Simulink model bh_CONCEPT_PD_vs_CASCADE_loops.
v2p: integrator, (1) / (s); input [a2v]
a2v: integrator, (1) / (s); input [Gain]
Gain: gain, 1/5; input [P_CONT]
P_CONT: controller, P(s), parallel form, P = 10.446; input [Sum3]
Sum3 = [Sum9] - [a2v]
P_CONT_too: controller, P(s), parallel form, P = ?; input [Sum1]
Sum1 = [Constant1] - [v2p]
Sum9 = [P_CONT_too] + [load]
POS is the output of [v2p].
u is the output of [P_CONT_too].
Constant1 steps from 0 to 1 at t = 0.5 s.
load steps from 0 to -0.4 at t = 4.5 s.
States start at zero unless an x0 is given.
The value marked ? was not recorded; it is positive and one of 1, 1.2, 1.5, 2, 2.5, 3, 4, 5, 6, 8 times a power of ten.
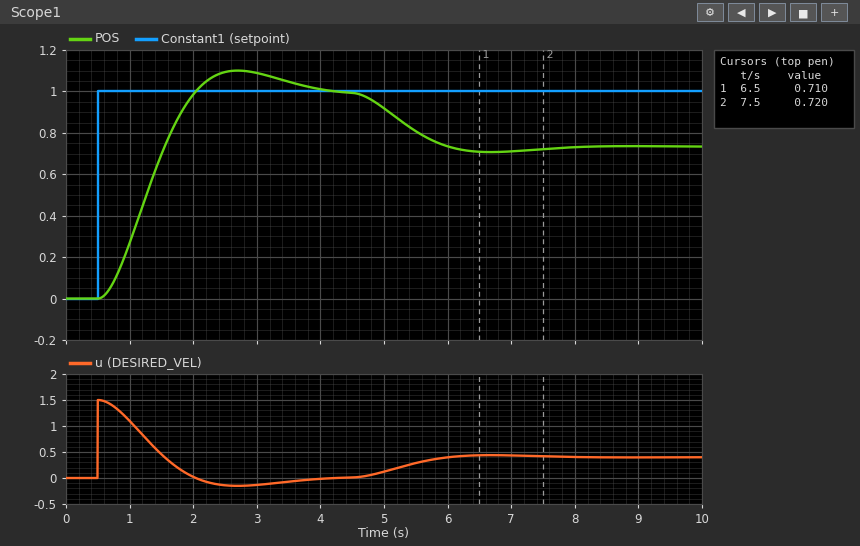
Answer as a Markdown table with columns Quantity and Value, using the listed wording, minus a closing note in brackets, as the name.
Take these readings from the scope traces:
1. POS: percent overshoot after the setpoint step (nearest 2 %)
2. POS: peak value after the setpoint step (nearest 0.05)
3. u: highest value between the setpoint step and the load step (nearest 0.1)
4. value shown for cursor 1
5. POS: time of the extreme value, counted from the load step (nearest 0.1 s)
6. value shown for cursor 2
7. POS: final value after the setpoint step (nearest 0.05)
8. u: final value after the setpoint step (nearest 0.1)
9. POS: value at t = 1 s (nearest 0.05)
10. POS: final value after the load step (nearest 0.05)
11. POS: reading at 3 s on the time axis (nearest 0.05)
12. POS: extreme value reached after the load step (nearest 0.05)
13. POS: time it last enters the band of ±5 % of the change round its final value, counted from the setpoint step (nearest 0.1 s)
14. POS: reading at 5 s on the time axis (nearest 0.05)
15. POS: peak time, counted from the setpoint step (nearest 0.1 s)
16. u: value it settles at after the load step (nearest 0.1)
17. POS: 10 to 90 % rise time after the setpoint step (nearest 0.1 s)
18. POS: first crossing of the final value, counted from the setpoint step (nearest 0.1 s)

| Quantity | Value |
|---|---|
| POS: percent overshoot after the setpoint step | 10 % |
| POS: peak value after the setpoint step | 1.10 |
| u: highest value between the setpoint step and the load step | 1.5 |
| value shown for cursor 1 | 0.710 |
| POS: time of the extreme value, counted from the load step | 2.2 s |
| value shown for cursor 2 | 0.720 |
| POS: final value after the setpoint step | 1.00 |
| u: final value after the setpoint step | 0.0 |
| POS: value at t = 1 s | 0.25 |
| POS: final value after the load step | 0.75 |
| POS: reading at 3 s on the time axis | 1.10 |
| POS: extreme value reached after the load step | 0.70 |
| POS: time it last enters the band of ±5 % of the change round its final value, counted from the setpoint step | 3.0 s |
| POS: reading at 5 s on the time axis | 0.90 |
| POS: peak time, counted from the setpoint step | 2.2 s |
| u: value it settles at after the load step | 0.4 |
| POS: 10 to 90 % rise time after the setpoint step | 1.0 s |
| POS: first crossing of the final value, counted from the setpoint step | 1.5 s |
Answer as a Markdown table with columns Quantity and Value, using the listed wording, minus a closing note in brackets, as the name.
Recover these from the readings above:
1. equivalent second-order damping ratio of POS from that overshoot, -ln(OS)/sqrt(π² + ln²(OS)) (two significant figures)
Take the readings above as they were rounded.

| Quantity | Value |
|---|---|
| equivalent second-order damping ratio of POS from that overshoot, -ln(OS)/sqrt(π² + ln²(OS)) | 0.59 |
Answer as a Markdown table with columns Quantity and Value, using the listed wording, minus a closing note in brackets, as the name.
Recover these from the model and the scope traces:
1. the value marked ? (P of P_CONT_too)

| Quantity | Value |
|---|---|
| the value marked ? | 1.5 |
